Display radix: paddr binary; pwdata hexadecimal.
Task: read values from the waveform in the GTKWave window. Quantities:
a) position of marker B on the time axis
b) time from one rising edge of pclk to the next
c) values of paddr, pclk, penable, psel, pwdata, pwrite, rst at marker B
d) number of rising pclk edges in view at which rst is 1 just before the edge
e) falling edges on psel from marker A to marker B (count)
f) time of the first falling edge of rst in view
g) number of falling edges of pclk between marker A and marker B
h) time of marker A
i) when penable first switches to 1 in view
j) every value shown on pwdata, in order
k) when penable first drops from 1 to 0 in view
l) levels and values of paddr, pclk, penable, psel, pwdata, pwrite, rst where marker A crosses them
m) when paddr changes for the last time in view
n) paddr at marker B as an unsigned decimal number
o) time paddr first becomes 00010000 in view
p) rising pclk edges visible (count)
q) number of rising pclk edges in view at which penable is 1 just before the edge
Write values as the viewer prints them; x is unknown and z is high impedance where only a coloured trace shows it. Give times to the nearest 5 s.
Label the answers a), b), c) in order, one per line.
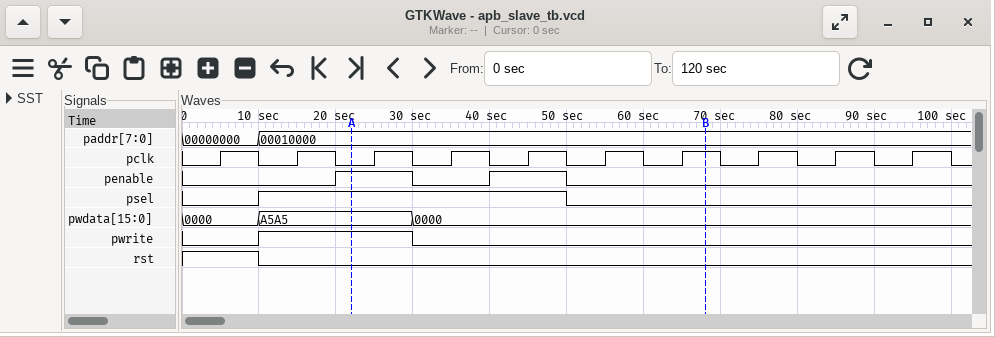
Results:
a) 70 s
b) 10 s
c) paddr=00010000, pclk=1, penable=0, psel=0, pwdata=0000, pwrite=0, rst=0
d) 1
e) 1
f) 10 s
g) 4
h) 20 s
i) 20 s
j) 0000, A5A5, 0000
k) 30 s
l) paddr=00010000, pclk=0, penable=1, psel=1, pwdata=A5A5, pwrite=1, rst=0
m) 10 s
n) 16
o) 10 s
p) 10
q) 2
